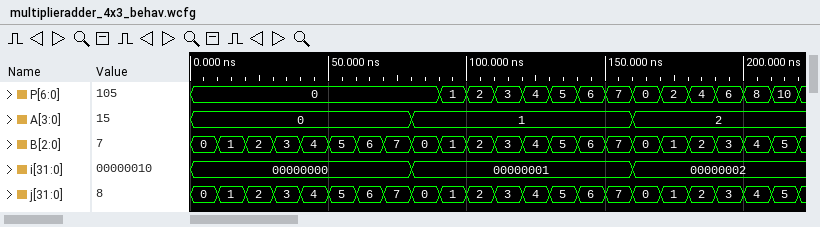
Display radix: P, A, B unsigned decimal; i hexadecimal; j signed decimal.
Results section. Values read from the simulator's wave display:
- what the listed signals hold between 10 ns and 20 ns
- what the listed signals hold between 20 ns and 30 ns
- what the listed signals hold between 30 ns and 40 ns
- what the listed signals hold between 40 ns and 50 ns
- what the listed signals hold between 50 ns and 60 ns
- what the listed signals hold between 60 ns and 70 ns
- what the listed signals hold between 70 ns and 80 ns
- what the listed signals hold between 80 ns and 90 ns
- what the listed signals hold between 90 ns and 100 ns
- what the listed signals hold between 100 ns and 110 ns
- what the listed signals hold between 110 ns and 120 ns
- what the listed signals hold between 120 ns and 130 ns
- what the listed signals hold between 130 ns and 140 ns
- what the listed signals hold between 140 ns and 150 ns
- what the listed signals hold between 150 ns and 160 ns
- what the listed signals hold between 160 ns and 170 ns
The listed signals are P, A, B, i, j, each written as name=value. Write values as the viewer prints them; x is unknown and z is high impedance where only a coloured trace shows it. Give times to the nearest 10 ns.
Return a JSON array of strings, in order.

["P=0, A=0, B=1, i=00000000, j=1", "P=0, A=0, B=2, i=00000000, j=2", "P=0, A=0, B=3, i=00000000, j=3", "P=0, A=0, B=4, i=00000000, j=4", "P=0, A=0, B=5, i=00000000, j=5", "P=0, A=0, B=6, i=00000000, j=6", "P=0, A=0, B=7, i=00000000, j=7", "P=0, A=1, B=0, i=00000001, j=0", "P=1, A=1, B=1, i=00000001, j=1", "P=2, A=1, B=2, i=00000001, j=2", "P=3, A=1, B=3, i=00000001, j=3", "P=4, A=1, B=4, i=00000001, j=4", "P=5, A=1, B=5, i=00000001, j=5", "P=6, A=1, B=6, i=00000001, j=6", "P=7, A=1, B=7, i=00000001, j=7", "P=0, A=2, B=0, i=00000002, j=0"]
